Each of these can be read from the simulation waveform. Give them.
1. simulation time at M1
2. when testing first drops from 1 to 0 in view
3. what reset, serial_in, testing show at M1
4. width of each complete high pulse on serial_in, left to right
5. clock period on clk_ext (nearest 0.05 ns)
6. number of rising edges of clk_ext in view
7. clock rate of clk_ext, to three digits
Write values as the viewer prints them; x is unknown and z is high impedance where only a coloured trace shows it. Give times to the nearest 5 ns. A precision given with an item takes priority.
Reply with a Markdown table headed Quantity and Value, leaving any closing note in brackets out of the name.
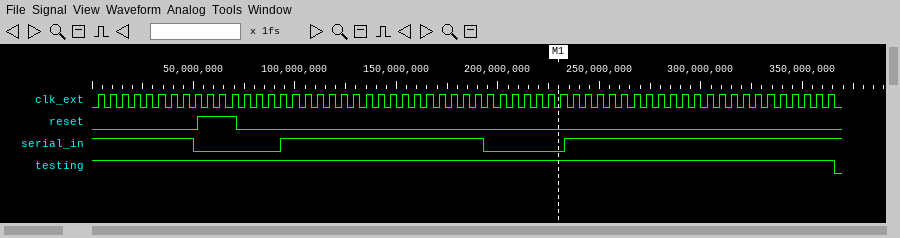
| Quantity | Value |
|---|---|
| simulation time at M1 | 230 ns |
| when testing first drops from 1 to 0 in view | 365 ns |
| what reset, serial_in, testing show at M1 | reset=0, serial_in=0, testing=1 |
| width of each complete high pulse on serial_in, left to right | 100 ns |
| clock period on clk_ext | 6 ns |
| number of rising edges of clk_ext in view | 61 |
| clock rate of clk_ext, to three digits | 167 MHz |
